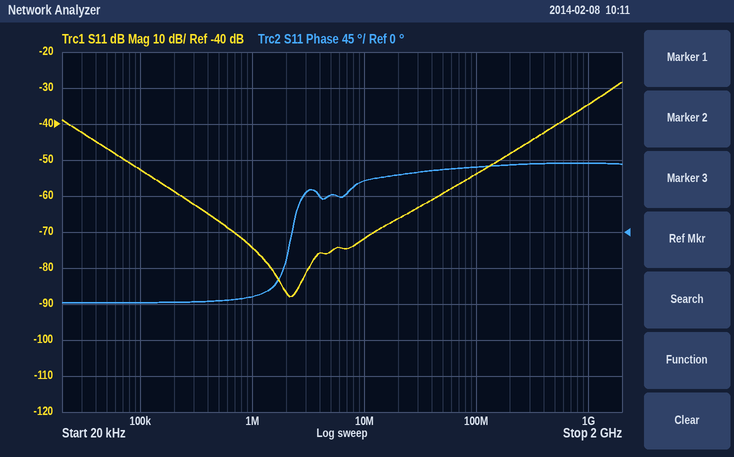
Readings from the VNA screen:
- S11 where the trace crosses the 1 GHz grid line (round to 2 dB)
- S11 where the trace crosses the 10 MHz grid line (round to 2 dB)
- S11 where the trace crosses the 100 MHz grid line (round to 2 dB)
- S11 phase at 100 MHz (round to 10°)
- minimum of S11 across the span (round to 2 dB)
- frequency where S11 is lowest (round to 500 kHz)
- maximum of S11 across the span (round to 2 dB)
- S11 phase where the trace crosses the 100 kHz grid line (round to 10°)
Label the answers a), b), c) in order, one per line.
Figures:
a) -34 dB
b) -72 dB
c) -54 dB
d) 80°
e) -88 dB
f) 2.0 MHz
g) -28 dB
h) -90°
